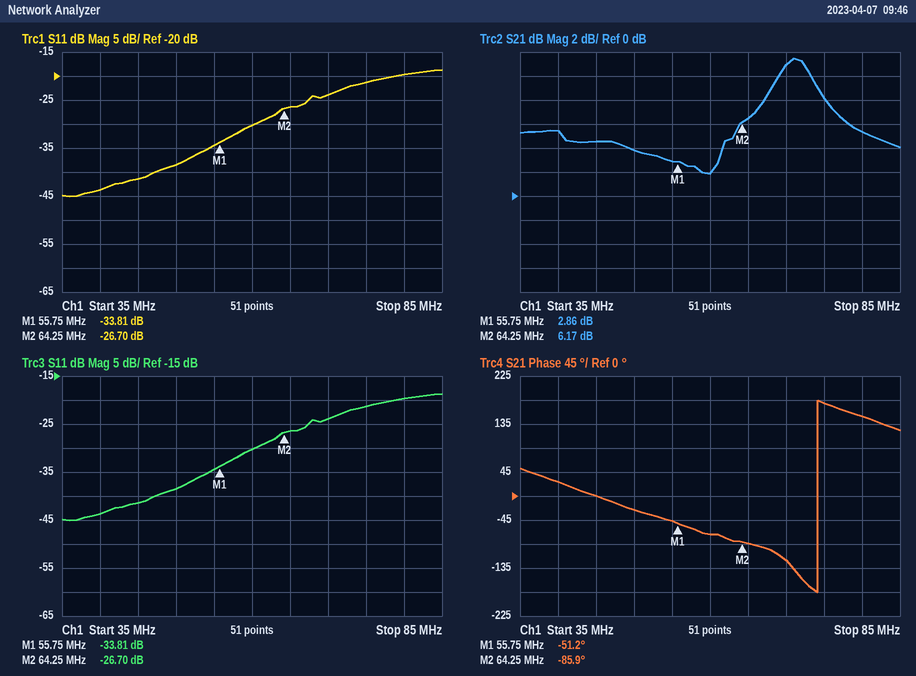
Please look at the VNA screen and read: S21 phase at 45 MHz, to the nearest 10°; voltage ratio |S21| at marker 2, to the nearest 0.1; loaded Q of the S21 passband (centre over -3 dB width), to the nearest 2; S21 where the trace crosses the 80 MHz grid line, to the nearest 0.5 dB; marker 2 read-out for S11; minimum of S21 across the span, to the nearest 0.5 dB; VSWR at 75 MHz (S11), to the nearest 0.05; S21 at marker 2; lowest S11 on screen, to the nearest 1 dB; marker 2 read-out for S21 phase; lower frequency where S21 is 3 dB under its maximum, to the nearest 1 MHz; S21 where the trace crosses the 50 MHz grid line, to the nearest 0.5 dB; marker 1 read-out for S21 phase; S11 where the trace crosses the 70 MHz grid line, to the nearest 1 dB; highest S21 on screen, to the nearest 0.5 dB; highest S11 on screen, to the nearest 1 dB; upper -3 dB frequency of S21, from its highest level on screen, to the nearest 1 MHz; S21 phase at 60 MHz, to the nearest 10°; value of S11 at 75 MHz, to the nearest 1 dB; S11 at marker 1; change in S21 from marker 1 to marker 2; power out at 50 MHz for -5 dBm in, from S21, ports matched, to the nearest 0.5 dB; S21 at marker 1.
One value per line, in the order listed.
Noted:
0°
2.0
10
5.5 dB
-26.70 dB
2.0 dB
1.20
6.17 dB
-45 dB
-85.9°
68 MHz
4.0 dB
-51.2°
-24 dB
11.5 dB
-19 dB
75 MHz
-70°
-21 dB
-33.81 dB
3.31 dB
-1.0 dBm
2.86 dB
